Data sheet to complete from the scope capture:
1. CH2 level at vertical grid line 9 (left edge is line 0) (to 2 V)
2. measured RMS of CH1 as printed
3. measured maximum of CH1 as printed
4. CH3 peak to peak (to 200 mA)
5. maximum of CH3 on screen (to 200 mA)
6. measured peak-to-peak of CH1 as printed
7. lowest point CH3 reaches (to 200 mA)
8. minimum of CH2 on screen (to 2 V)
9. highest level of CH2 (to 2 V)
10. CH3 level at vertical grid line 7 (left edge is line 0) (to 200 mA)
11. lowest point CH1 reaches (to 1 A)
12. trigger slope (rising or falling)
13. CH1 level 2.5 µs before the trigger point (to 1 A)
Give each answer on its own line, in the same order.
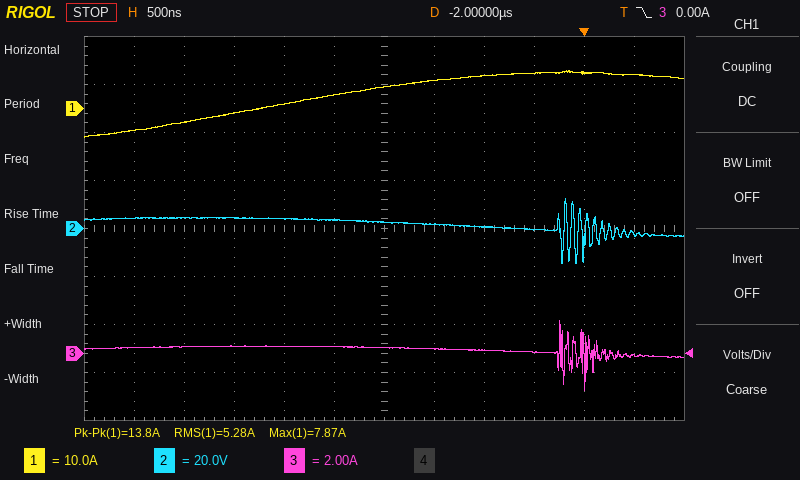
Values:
0 V
5.28 A
7.87 A
3.0 A
1.4 A
13.8 A
-1.6 A
-14 V
12 V
200 mA
-6 A
falling
3 A
